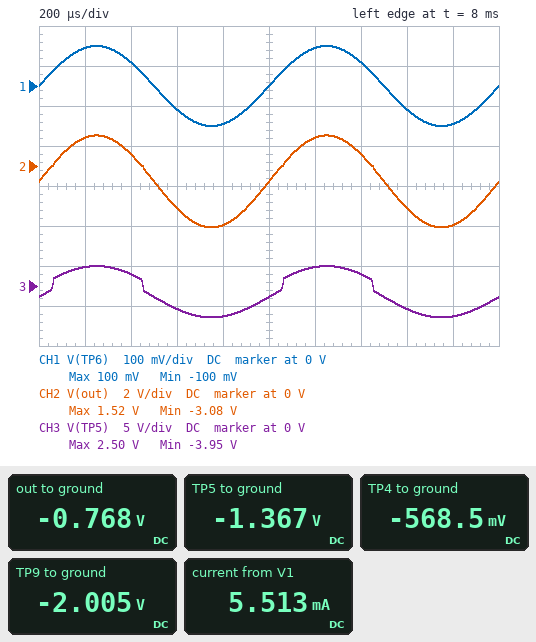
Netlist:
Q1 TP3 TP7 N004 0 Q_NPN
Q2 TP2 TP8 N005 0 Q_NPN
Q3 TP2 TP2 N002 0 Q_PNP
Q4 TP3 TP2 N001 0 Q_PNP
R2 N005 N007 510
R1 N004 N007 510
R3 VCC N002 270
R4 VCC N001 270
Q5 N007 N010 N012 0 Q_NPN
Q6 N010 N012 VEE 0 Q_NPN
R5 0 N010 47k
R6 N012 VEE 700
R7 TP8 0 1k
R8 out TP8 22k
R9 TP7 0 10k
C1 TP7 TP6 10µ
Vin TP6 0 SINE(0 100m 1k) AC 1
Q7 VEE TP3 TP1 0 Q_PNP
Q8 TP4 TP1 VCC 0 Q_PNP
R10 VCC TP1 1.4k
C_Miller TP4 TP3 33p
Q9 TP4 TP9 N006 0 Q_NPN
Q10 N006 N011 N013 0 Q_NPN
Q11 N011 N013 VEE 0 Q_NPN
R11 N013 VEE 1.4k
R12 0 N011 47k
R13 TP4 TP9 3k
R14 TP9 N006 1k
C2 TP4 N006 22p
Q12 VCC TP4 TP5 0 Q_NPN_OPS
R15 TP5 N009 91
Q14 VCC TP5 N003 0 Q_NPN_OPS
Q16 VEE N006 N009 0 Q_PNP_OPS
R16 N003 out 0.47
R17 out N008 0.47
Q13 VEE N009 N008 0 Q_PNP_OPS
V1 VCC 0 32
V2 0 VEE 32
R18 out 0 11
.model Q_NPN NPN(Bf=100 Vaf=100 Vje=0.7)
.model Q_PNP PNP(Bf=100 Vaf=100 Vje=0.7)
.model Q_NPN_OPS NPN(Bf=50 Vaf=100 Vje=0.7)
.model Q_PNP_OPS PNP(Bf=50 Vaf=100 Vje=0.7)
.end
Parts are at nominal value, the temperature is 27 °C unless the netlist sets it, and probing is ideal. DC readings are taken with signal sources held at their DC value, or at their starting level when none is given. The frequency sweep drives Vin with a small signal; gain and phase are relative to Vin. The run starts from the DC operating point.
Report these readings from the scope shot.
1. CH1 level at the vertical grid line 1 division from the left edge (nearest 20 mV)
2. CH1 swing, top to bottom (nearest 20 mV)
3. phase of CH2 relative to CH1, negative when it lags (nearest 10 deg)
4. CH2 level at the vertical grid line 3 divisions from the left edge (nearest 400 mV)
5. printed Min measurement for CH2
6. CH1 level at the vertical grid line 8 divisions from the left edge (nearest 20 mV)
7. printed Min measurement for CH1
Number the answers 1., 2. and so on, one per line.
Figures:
1. 100 mV
2. 200 mV
3. 0 deg
4. -2.0 V
5. -3.08 V
6. -60 mV
7. -100 mV
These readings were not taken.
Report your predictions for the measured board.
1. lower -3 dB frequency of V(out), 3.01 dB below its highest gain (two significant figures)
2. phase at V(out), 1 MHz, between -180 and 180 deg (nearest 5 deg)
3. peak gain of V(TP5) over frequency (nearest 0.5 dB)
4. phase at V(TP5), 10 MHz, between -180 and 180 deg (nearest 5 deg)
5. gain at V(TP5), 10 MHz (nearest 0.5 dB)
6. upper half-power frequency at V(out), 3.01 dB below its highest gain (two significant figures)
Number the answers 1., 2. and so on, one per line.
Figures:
1. 1.6 Hz
2. -70 deg
3. 28.5 dB
4. -95 deg
5. -1.5 dB
6. 320 kHz
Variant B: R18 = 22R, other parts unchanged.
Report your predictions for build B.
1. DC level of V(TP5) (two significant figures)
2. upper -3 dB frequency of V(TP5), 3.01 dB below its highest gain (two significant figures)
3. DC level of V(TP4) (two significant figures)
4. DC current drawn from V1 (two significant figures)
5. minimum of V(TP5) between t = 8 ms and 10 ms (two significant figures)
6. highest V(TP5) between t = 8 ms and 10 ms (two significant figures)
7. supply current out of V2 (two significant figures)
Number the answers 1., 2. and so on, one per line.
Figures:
1. -1.3 V
2. 340 kHz
3. -510 mV
4. 5.7 mA
5. -3.8 V
6. 2.4 V
7. 42 mA
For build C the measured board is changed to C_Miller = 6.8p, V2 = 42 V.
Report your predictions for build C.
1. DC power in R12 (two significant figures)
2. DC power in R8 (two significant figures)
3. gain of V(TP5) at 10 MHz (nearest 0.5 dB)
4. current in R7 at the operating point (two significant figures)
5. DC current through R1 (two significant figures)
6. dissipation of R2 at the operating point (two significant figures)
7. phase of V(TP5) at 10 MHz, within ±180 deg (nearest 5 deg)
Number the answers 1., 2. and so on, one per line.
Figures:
1. 35 mW
2. 25 µW
3. 12.0 dB
4. 38 µA
5. 550 µA
6. 160 µW
7. -80 deg
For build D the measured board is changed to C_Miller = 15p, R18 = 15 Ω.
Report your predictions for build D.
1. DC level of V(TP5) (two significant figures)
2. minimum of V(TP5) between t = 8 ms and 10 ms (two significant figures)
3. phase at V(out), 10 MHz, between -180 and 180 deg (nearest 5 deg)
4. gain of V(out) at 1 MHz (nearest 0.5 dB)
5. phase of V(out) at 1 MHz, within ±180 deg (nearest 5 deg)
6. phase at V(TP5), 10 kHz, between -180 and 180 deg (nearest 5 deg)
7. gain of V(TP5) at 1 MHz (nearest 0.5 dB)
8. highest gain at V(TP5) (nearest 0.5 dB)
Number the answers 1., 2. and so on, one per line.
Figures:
1. -1.3 V
2. -3.8 V
3. -90 deg
4. 22.5 dB
5. -55 deg
6. 0 deg
7. 23.5 dB
8. 28.0 dB
